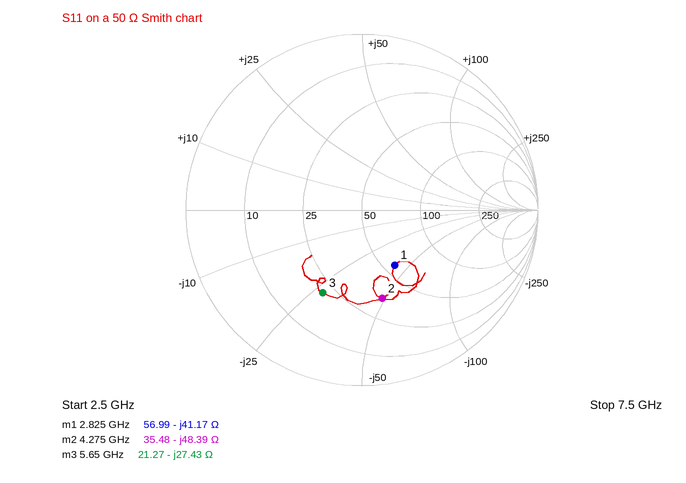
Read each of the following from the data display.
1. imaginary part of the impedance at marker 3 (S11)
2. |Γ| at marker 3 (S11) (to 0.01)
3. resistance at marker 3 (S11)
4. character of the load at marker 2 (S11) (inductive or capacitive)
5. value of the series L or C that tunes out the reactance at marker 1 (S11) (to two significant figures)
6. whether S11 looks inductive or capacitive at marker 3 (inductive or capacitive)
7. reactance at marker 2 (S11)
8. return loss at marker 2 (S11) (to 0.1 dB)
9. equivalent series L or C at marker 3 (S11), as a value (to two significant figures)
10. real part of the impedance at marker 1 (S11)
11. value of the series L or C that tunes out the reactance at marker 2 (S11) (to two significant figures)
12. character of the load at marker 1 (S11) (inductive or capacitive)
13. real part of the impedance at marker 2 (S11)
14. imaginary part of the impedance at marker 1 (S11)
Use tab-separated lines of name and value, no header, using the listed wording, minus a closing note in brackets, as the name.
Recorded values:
imaginary part of the impedance at marker 3	-27.43 Ω
|Γ| at marker 3 (S11)	0.52
resistance at marker 3	21.27 Ω
character of the load at marker 2 (S11)	capacitive
value of the series L or C that tunes out the reactance at marker 1 (S11)	2.3 nH
whether S11 looks inductive or capacitive at marker 3	capacitive
reactance at marker 2	-48.39 Ω
return loss at marker 2 (S11)	5.8 dB
equivalent series L or C at marker 3 (S11), as a value	1.0 pF
real part of the impedance at marker 1	56.99 Ω
value of the series L or C that tunes out the reactance at marker 2 (S11)	1.8 nH
character of the load at marker 1 (S11)	capacitive
real part of the impedance at marker 2	35.48 Ω
imaginary part of the impedance at marker 1	-41.17 Ω
